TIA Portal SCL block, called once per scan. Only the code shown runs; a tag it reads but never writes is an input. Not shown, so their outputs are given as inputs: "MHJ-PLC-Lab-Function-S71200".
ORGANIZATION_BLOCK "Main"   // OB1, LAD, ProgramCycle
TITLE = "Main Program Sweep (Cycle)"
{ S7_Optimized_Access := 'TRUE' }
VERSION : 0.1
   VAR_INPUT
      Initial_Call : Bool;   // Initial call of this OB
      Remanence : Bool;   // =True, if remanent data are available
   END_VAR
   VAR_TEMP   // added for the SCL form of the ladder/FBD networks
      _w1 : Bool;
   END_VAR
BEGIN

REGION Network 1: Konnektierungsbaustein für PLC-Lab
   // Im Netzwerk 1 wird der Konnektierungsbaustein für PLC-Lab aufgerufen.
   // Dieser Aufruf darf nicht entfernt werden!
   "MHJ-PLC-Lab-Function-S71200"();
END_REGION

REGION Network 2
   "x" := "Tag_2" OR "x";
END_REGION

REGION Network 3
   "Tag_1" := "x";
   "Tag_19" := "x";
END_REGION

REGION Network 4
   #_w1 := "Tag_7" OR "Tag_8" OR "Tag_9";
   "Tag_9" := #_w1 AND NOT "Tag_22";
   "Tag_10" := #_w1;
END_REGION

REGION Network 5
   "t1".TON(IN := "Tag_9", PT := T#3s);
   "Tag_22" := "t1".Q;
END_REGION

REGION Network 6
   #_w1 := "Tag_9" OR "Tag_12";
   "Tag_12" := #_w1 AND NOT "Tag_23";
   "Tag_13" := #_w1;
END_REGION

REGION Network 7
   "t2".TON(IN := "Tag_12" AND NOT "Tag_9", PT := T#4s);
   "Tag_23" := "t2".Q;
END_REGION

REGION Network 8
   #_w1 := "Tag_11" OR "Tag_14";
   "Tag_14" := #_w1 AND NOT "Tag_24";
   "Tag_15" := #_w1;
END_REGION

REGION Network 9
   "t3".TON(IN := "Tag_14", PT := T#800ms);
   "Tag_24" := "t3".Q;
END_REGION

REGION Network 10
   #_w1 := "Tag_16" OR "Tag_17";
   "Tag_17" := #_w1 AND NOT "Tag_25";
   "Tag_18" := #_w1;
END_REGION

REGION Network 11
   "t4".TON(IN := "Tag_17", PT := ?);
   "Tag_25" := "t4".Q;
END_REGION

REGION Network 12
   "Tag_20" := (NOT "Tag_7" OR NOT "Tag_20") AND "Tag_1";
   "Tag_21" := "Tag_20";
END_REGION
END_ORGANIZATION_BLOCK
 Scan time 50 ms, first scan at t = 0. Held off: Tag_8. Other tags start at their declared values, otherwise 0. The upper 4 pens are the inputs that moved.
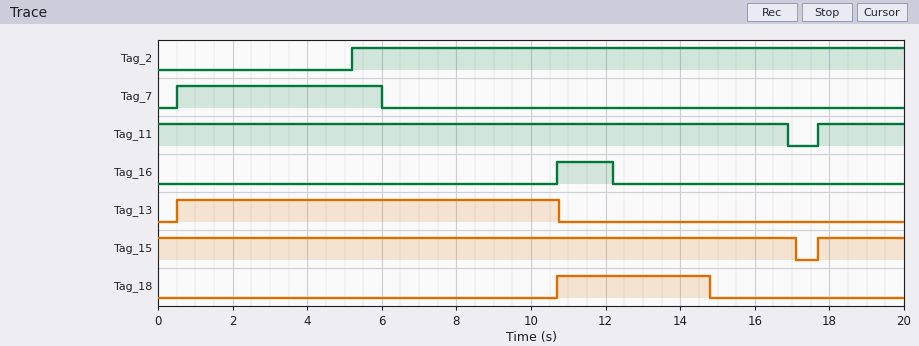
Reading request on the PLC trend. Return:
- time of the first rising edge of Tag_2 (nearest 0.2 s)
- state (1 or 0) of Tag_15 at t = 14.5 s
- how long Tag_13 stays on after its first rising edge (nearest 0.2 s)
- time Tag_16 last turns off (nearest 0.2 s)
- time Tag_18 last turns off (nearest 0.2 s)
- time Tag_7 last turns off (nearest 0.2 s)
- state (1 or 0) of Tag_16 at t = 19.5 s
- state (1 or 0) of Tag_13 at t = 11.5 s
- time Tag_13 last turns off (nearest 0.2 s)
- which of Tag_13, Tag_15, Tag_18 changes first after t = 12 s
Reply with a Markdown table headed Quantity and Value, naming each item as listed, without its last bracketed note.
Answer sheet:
| Quantity | Value |
|---|---|
| time of the first rising edge of Tag_2 | 5.2 s |
| state (1 or 0) of Tag_15 at t = 14.5 s | 1 |
| how long Tag_13 stays on after its first rising edge | 10.2 s |
| time Tag_16 last turns off | 12.2 s |
| time Tag_18 last turns off | 14.8 s |
| time Tag_7 last turns off | 6.0 s |
| state (1 or 0) of Tag_16 at t = 19.5 s | 0 |
| state (1 or 0) of Tag_13 at t = 11.5 s | 0 |
| time Tag_13 last turns off | 10.8 s |
| which of Tag_13, Tag_15, Tag_18 changes first after t = 12 s | Tag_18 |
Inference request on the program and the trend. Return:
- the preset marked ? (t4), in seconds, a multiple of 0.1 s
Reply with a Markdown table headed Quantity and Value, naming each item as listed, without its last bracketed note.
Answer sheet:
| Quantity | Value |
|---|---|
| the preset marked ? (t4), in seconds, a multiple of 0.1 s | 4.0 s |
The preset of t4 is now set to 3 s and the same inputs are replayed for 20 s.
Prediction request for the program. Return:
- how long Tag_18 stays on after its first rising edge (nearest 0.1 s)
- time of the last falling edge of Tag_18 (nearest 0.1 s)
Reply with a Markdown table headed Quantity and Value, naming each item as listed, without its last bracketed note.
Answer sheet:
| Quantity | Value |
|---|---|
| how long Tag_18 stays on after its first rising edge | 3.1 s |
| time of the last falling edge of Tag_18 | 13.8 s |
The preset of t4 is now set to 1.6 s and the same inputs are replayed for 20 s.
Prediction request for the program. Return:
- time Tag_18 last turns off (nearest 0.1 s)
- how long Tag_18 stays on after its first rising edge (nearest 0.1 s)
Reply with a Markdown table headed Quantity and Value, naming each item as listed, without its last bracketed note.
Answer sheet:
| Quantity | Value |
|---|---|
| time Tag_18 last turns off | 12.4 s |
| how long Tag_18 stays on after its first rising edge | 1.7 s |
